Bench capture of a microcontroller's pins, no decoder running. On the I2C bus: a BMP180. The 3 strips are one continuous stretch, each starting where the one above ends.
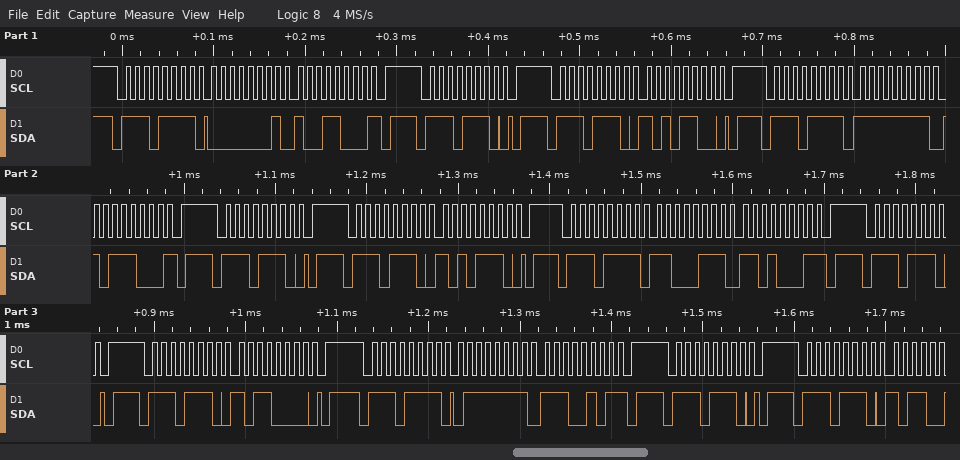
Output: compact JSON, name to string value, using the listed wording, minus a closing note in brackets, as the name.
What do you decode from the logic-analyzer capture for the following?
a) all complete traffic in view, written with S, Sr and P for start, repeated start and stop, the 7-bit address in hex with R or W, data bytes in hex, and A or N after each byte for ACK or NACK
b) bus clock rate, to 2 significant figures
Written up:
{"all complete traffic in view, written with S, Sr and P for start, repeated start and stop, the 7-bit address in hex with R or W, data bytes in hex, and A or N after each byte for ACK or NACK": "S 77R A 01 A 98 N P S 77W A P S 77W A AC A P S 77R A FF A B8 N P S 77W A P S 77W A AE A P S 77R A C7 A D1 N P S 77W A P S 77W A B0 A P S 77R A 7F A E5 N P S 77W A P S 77W A", "bus clock rate, to 2 significant figures": "100 kHz"}
